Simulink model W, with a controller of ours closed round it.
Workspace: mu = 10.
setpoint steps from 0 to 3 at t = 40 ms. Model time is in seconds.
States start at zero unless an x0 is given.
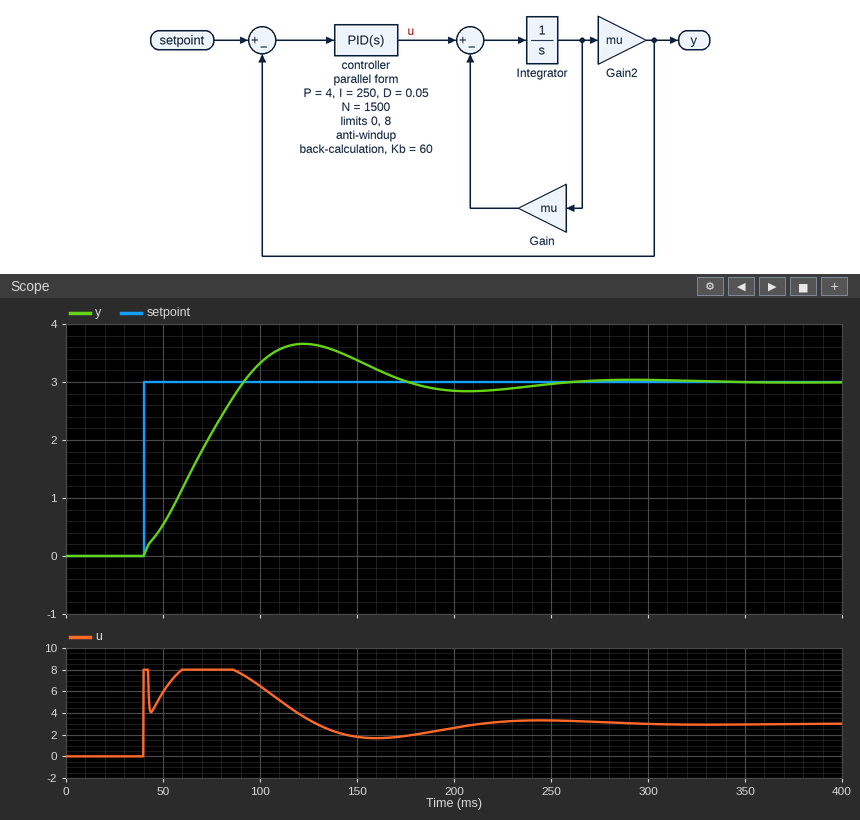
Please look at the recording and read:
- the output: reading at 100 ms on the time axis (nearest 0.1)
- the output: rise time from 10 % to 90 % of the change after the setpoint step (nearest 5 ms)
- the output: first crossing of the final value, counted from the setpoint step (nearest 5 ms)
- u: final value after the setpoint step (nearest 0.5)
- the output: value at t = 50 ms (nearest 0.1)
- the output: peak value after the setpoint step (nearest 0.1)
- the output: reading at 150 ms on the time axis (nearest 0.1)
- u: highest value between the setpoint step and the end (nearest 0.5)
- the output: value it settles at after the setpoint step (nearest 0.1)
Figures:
3.3
40 ms
50 ms
3.0
0.5
3.7
3.4
8.0
3.0
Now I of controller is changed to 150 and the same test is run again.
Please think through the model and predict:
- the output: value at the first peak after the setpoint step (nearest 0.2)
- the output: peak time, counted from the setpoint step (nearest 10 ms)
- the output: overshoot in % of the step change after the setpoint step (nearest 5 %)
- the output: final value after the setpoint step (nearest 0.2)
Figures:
3.4
110 ms
15 %
3.0
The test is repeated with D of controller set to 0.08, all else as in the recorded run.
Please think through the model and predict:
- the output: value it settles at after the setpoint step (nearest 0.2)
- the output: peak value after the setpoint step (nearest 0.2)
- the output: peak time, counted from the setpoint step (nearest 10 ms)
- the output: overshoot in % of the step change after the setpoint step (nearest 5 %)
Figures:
3.0
3.8
90 ms
25 %
